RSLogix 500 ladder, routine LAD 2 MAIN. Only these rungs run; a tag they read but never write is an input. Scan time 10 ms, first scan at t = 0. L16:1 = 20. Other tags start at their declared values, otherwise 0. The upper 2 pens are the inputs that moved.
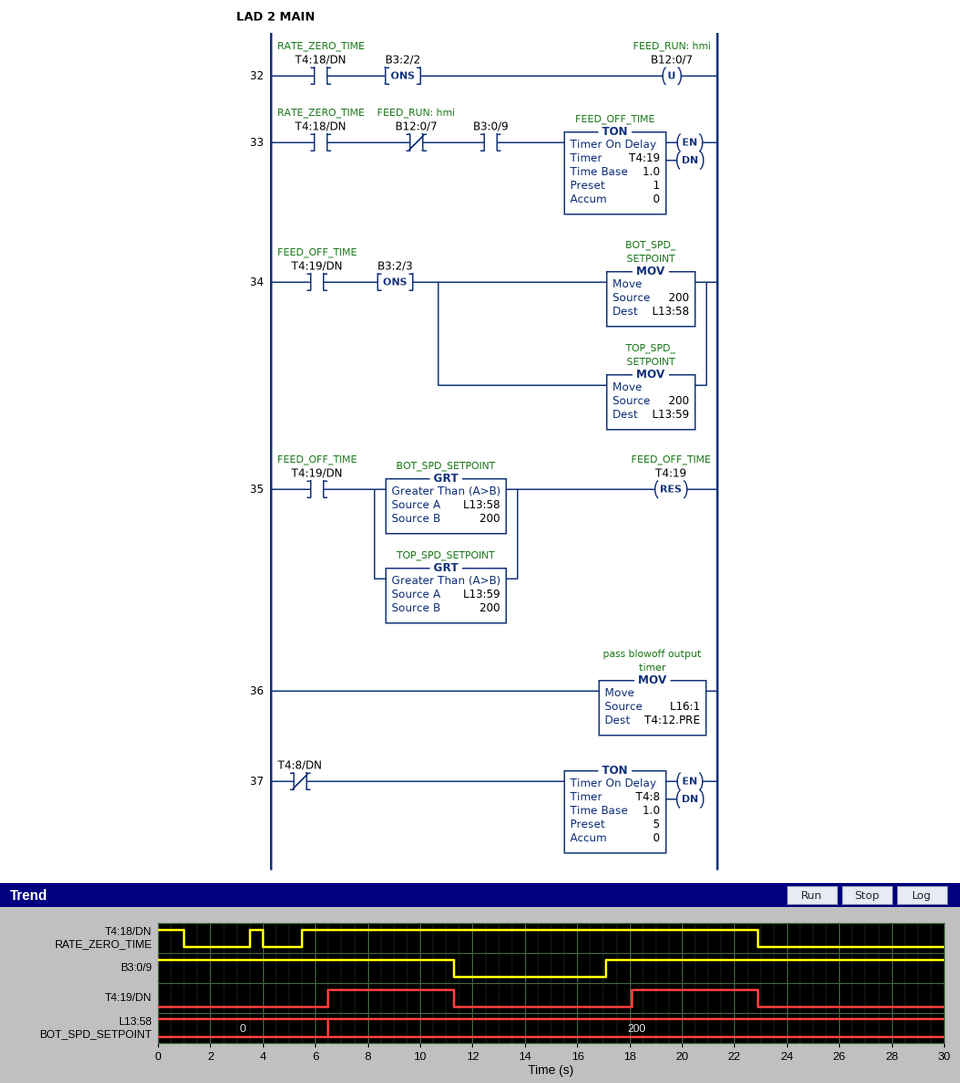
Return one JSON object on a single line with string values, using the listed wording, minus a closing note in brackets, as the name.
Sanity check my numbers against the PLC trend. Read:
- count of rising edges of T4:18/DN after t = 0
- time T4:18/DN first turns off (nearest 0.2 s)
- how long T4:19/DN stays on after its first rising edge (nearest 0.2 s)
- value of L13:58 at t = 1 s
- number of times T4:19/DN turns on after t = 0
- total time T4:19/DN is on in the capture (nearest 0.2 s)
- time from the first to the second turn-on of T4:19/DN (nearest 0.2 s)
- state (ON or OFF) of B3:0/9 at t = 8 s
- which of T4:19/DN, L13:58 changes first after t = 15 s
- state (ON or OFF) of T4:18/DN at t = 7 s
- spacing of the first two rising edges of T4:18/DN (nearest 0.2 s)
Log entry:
{"count of rising edges of T4:18/DN after t = 0": "2", "time T4:18/DN first turns off": "1.0 s", "how long T4:19/DN stays on after its first rising edge": "4.8 s", "value of L13:58 at t = 1 s": "0", "number of times T4:19/DN turns on after t = 0": "2", "total time T4:19/DN is on in the capture": "9.6 s", "time from the first to the second turn-on of T4:19/DN": "11.6 s", "state (ON or OFF) of B3:0/9 at t = 8 s": "ON", "which of T4:19/DN, L13:58 changes first after t = 15 s": "T4:19/DN", "state (ON or OFF) of T4:18/DN at t = 7 s": "ON", "spacing of the first two rising edges of T4:18/DN": "2.0 s"}
